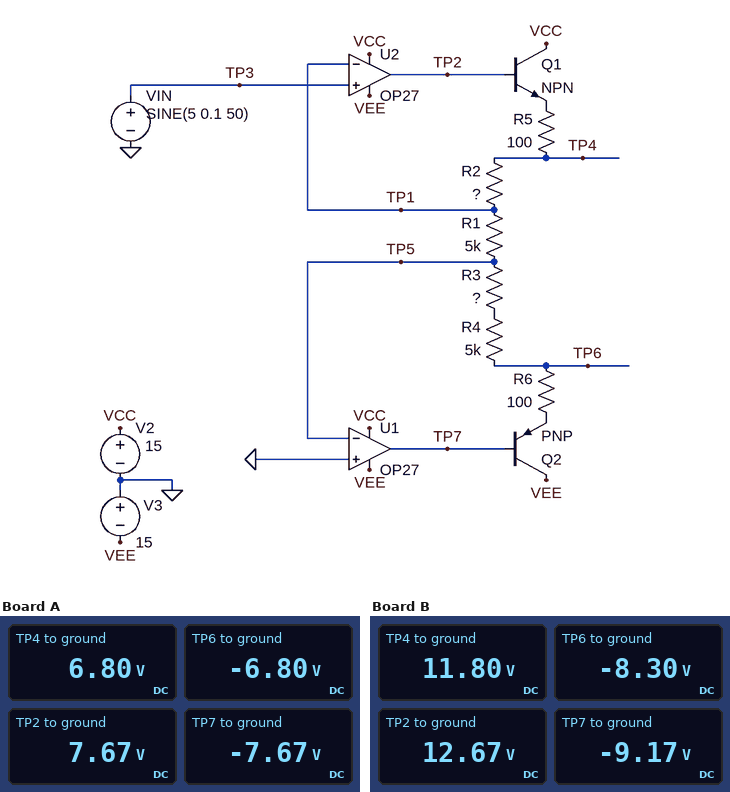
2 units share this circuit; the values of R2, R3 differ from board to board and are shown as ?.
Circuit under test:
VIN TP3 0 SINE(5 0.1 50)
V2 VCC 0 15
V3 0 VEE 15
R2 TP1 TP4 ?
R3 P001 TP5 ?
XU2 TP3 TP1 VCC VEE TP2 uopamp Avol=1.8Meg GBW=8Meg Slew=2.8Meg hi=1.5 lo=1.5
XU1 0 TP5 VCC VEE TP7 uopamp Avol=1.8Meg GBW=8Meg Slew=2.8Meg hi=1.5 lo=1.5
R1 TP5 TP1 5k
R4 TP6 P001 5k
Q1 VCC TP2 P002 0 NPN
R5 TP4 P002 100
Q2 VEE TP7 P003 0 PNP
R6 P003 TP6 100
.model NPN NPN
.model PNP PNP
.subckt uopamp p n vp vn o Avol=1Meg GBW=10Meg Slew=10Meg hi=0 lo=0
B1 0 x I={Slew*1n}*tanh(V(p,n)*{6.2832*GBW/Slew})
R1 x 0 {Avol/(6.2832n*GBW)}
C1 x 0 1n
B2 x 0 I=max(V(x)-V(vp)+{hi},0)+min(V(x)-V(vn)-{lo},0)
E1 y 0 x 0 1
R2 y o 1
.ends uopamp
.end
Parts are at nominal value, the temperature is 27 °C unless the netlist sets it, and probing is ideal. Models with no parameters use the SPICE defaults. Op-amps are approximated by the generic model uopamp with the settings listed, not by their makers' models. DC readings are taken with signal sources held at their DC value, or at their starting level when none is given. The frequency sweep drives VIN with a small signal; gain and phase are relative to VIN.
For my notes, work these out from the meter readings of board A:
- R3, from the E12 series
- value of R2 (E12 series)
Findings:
1.8 kΩ
1.8 kΩ
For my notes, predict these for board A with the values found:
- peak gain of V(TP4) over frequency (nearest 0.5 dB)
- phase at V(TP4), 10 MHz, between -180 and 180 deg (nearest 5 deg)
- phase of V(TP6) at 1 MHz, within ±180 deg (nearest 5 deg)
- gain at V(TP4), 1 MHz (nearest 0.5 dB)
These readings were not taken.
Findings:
2.5 dB
-55 deg
155 deg
2.5 dB
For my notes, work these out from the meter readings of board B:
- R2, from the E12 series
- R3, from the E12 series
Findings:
6.8 kΩ
3.3 kΩ
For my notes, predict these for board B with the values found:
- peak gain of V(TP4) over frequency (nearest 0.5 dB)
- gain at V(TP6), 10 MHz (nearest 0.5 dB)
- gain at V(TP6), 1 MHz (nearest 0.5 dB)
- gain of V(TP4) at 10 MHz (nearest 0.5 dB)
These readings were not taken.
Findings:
7.5 dB
-14.0 dB
3.5 dB
-3.5 dB
